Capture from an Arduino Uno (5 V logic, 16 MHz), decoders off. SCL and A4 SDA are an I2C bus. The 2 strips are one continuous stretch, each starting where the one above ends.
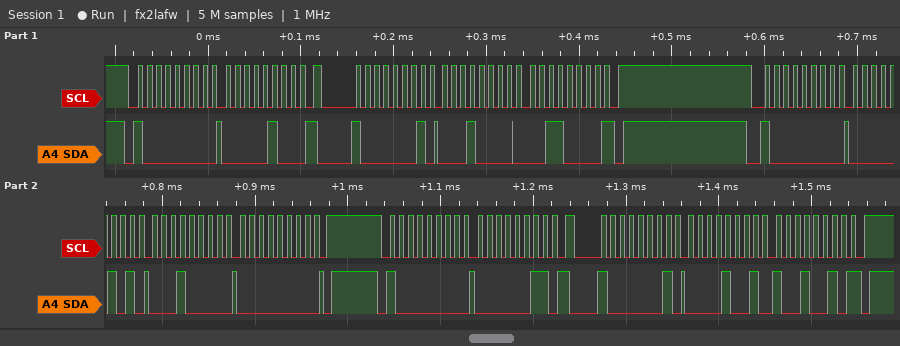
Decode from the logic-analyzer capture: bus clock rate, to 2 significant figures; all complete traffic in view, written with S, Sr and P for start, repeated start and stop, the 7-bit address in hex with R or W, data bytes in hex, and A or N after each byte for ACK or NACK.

100 kHz
S 40W A 04 A Sr 40R A 10 A 30 N P S 40W A 05 A 10 A 00 A P S 40W A 03 A Sr 40R A 09 A 92 N P
